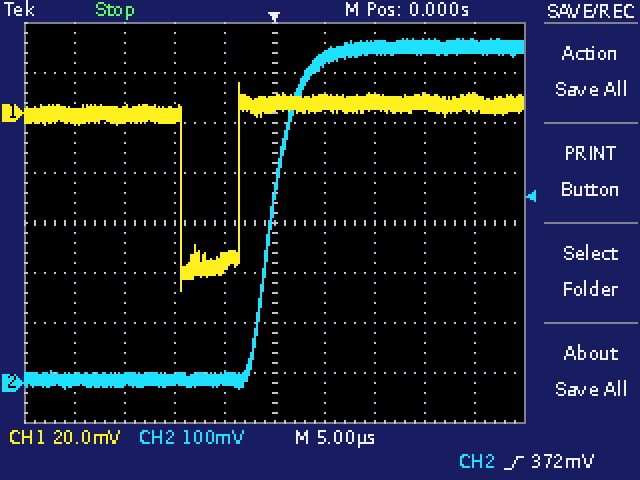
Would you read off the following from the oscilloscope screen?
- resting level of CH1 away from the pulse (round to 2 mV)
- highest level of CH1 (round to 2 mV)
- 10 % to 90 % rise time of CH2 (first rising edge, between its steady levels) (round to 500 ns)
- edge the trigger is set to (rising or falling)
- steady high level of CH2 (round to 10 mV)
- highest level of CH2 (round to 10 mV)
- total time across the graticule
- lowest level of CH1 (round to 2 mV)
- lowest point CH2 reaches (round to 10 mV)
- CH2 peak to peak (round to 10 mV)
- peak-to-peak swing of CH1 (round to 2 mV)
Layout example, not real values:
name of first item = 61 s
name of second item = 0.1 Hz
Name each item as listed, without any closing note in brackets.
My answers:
resting level of CH1 away from the pulse = 4 mV
highest level of CH1 = 12 mV
10 % to 90 % rise time of CH2 (first rising edge, between its steady levels) = 5.0 µs
edge the trigger is set to = rising
steady high level of CH2 = 670 mV
highest level of CH2 = 690 mV
total time across the graticule = 50 µs
lowest level of CH1 = -72 mV
lowest point CH2 reaches = -10 mV
CH2 peak to peak = 700 mV
peak-to-peak swing of CH1 = 84 mV
